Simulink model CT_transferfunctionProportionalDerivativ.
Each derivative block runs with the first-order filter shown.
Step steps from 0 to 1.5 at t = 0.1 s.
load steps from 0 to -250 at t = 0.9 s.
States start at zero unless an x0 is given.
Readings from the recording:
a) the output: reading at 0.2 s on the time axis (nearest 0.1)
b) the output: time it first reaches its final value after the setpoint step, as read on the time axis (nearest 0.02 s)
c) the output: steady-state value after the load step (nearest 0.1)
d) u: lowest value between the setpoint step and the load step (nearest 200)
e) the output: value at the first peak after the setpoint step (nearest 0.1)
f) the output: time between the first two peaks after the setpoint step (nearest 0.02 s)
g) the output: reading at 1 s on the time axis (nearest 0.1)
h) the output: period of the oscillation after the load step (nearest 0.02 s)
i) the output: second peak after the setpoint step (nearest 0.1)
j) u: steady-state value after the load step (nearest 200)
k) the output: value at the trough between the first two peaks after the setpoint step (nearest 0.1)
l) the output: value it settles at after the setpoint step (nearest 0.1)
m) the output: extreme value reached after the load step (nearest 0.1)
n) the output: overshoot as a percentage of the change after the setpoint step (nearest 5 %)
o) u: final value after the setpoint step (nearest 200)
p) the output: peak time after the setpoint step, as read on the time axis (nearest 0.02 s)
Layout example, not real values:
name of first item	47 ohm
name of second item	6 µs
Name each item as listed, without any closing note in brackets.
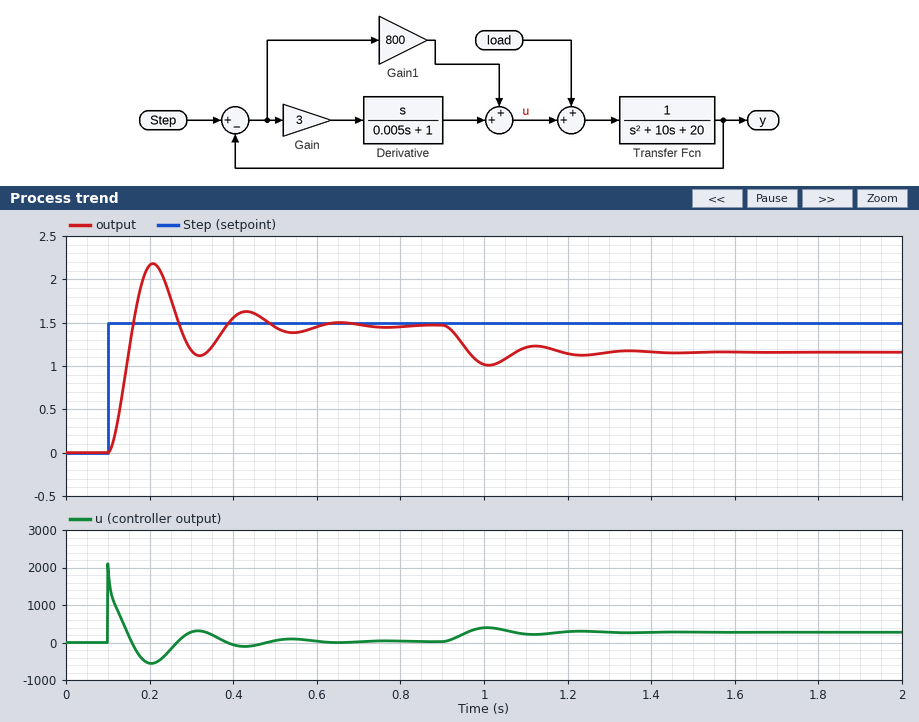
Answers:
the output: reading at 0.2 s on the time axis	2.2
the output: time it first reaches its final value after the setpoint step, as read on the time axis	0.16 s
the output: steady-state value after the load step	1.2
u: lowest value between the setpoint step and the load step	-600
the output: value at the first peak after the setpoint step	2.2
the output: time between the first two peaks after the setpoint step	0.22 s
the output: reading at 1 s on the time axis	1.0
the output: period of the oscillation after the load step	0.22 s
the output: second peak after the setpoint step	1.6
u: steady-state value after the load step	200
the output: value at the trough between the first two peaks after the setpoint step	1.1
the output: value it settles at after the setpoint step	1.5
the output: extreme value reached after the load step	1.0
the output: overshoot as a percentage of the change after the setpoint step	50 %
u: final value after the setpoint step	0
the output: peak time after the setpoint step, as read on the time axis	0.20 s
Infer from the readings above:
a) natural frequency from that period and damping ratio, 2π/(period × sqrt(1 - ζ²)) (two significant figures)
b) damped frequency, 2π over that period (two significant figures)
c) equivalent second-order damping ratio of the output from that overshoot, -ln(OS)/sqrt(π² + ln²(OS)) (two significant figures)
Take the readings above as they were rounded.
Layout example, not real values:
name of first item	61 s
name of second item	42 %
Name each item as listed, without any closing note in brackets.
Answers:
natural frequency from that period and damping ratio, 2π/(period × sqrt(1 - ζ²))	29 rad/s
damped frequency, 2π over that period	29 rad/s
equivalent second-order damping ratio of the output from that overshoot, -ln(OS)/sqrt(π² + ln²(OS))	0.22
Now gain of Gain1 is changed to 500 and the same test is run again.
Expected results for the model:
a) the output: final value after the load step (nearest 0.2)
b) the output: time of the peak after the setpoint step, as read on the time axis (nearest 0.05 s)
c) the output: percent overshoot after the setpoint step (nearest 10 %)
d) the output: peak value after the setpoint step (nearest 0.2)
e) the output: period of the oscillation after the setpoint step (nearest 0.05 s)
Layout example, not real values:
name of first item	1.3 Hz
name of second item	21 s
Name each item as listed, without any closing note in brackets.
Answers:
the output: final value after the load step	1.0
the output: time of the peak after the setpoint step, as read on the time axis	0.25 s
the output: percent overshoot after the setpoint step	40 %
the output: peak value after the setpoint step	2.0
the output: period of the oscillation after the setpoint step	0.30 s
